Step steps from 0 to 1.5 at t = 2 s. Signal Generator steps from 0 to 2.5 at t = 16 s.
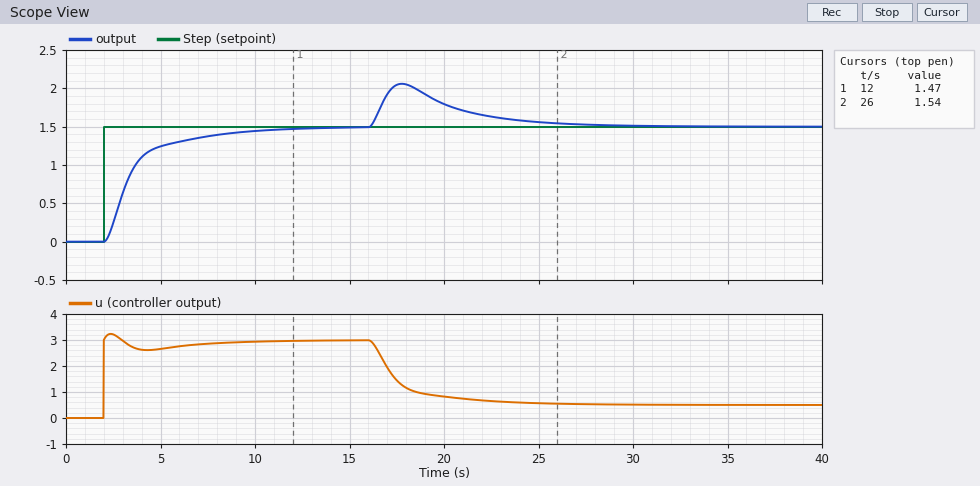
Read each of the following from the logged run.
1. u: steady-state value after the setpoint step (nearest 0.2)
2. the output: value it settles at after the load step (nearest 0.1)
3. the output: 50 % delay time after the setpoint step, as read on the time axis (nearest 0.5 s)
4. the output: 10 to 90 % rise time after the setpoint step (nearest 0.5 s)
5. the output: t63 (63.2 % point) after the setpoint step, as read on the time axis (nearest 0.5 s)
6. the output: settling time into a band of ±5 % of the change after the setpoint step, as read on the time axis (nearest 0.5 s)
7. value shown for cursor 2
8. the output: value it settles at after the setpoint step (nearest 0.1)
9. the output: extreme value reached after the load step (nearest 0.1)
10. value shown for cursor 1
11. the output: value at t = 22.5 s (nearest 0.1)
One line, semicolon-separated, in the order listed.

3.0; 1.5; 3.0 s; 4.5 s; 3.5 s; 9.0 s; 1.54; 1.5; 2.1; 1.47; 1.6
